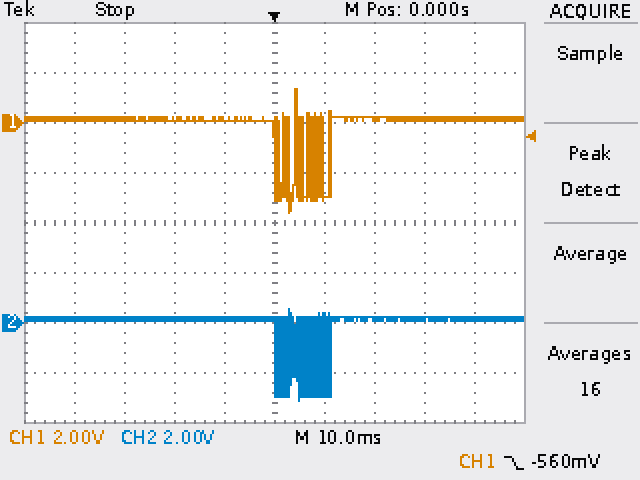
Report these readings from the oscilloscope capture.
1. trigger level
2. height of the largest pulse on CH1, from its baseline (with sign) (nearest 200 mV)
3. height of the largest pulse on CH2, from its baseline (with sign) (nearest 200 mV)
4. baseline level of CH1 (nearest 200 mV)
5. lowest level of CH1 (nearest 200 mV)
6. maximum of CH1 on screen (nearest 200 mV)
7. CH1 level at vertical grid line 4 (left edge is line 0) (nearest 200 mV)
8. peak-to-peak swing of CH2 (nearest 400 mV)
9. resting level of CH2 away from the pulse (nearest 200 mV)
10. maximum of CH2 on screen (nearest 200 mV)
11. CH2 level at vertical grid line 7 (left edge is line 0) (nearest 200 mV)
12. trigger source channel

-560 mV
-3.8 V
-3.2 V
200 mV
-3.6 V
1.4 V
200 mV
3.6 V
200 mV
600 mV
200 mV
CH1
